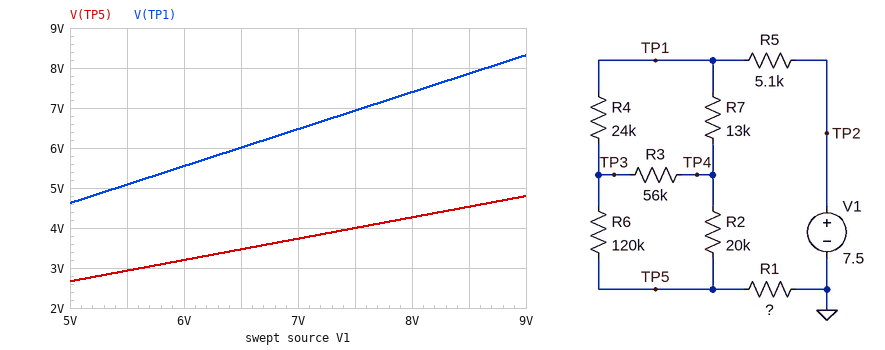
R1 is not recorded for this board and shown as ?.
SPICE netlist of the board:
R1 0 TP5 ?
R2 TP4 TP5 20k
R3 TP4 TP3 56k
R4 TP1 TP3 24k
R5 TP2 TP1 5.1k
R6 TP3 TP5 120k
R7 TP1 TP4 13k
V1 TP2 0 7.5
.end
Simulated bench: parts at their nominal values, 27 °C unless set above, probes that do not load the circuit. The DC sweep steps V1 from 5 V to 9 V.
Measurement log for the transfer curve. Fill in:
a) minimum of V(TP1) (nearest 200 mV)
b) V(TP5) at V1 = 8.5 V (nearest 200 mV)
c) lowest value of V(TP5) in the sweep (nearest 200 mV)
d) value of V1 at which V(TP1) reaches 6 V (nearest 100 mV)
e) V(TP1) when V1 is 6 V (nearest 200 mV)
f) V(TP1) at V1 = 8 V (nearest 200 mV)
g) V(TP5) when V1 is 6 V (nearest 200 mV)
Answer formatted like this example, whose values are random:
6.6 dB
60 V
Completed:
4.6 V
4.6 V
2.6 V
6.5 V
5.6 V
7.4 V
3.2 V
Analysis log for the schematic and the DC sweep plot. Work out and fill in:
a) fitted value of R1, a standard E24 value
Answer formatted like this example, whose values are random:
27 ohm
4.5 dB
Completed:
36 kΩ
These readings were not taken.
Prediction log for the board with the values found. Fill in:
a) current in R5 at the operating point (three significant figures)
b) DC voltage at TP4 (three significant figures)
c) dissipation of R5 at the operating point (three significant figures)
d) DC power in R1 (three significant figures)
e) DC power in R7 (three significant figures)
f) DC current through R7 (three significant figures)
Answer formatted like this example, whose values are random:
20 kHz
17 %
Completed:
111 µA
5.84 V
62.9 µW
444 µW
91.9 µW
84.1 µA
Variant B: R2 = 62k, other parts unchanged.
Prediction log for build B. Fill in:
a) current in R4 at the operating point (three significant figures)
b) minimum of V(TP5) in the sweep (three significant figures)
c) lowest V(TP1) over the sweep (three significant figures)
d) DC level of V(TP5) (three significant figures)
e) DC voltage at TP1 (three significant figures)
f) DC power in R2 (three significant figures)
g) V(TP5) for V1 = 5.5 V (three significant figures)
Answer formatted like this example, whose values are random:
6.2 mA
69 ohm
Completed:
28.7 µA
1.99 V
4.72 V
2.99 V
7.08 V
185 µW
2.19 V
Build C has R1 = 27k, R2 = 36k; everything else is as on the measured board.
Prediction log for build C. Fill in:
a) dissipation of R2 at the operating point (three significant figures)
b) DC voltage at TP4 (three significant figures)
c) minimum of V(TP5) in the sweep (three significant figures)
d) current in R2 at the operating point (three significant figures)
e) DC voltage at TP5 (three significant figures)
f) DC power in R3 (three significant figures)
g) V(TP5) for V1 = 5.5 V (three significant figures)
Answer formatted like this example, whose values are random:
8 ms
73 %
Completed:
245 µW
5.93 V
1.97 V
82.6 µA
2.96 V
1.18 µW
2.17 V
